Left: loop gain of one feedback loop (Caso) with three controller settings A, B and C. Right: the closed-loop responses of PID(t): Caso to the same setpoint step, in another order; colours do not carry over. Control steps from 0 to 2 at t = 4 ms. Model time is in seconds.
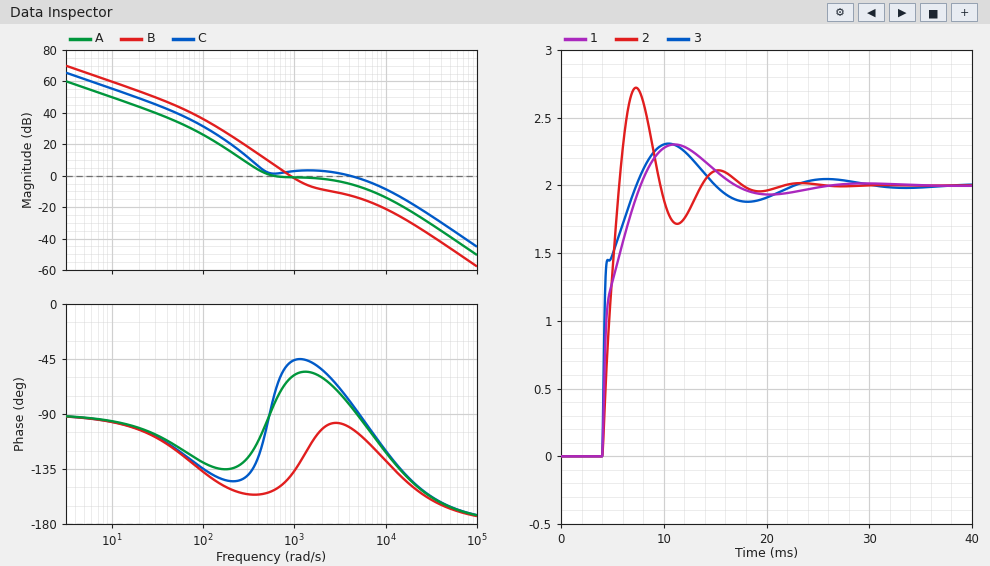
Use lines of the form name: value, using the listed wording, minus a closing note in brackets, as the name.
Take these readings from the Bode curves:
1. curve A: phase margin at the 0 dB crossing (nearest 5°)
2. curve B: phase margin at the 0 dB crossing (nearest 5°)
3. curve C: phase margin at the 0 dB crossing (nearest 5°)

curve A: phase margin at the 0 dB crossing: 95°
curve B: phase margin at the 0 dB crossing: 40°
curve C: phase margin at the 0 dB crossing: 100°
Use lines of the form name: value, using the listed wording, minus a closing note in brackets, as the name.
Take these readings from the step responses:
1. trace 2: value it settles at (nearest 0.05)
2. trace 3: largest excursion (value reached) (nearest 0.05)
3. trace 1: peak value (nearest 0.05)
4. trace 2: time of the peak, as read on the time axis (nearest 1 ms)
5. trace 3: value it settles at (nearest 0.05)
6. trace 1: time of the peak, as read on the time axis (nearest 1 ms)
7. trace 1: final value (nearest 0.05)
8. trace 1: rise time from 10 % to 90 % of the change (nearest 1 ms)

trace 2: value it settles at: 2.00
trace 3: largest excursion (value reached): 2.30
trace 1: peak value: 2.30
trace 2: time of the peak, as read on the time axis: 7 ms
trace 3: value it settles at: 2.00
trace 1: time of the peak, as read on the time axis: 11 ms
trace 1: final value: 2.00
trace 1: rise time from 10 % to 90 % of the change: 3 ms
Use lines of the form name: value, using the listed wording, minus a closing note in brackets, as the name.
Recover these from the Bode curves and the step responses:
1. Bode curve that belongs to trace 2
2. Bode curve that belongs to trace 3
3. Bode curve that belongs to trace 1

Bode curve that belongs to trace 2: B
Bode curve that belongs to trace 3: C
Bode curve that belongs to trace 1: A
